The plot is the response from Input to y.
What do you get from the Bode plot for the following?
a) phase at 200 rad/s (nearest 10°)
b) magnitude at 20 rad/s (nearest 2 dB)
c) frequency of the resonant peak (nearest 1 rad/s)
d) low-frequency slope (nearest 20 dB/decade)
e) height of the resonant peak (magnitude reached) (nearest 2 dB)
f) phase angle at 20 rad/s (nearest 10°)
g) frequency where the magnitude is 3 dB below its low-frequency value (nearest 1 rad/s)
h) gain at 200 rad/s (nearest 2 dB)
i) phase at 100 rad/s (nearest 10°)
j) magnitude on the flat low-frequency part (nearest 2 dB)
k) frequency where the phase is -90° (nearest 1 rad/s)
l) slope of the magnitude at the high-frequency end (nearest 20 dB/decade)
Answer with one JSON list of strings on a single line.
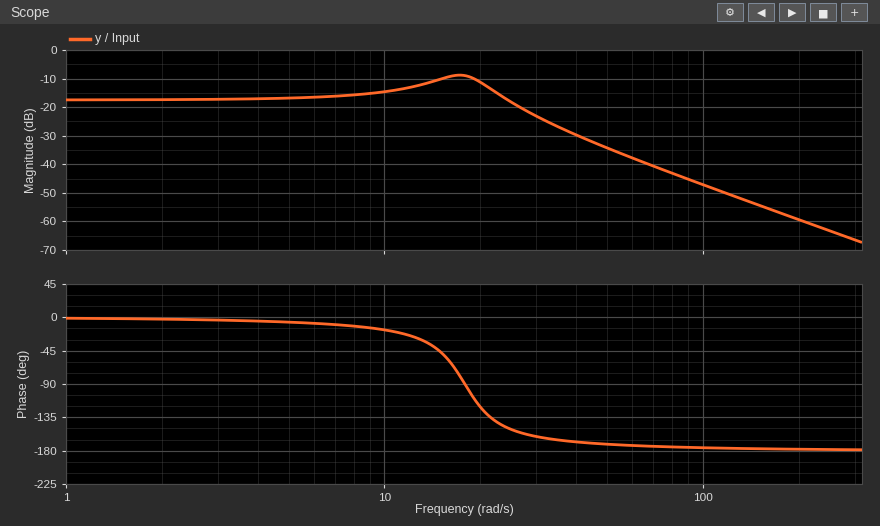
["-180°", "-12 dB", "17 rad/s", "0 dB/decade", "-8 dB", "-120°", "27 rad/s", "-60 dB", "-180°", "-18 dB", "18 rad/s", "-40 dB/decade"]
